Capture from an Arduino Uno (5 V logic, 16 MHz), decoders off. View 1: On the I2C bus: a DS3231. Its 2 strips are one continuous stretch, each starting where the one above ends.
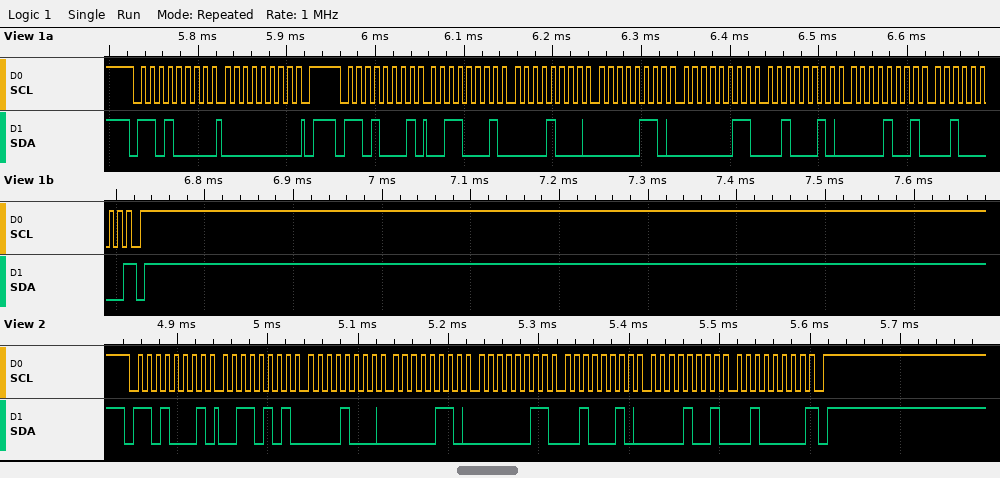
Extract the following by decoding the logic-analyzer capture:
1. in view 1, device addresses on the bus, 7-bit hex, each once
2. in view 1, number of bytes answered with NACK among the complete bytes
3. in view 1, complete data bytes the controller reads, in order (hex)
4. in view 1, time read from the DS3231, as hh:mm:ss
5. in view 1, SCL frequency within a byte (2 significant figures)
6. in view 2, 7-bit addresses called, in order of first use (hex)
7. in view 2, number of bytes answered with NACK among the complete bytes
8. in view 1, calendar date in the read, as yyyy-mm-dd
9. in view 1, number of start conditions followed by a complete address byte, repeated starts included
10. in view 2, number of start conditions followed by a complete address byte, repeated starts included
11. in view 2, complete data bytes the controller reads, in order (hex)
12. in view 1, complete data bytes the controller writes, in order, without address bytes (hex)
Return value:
0x68
1
31 08 06 03 22 09 20
06:08:31
100 kHz
0x68
1
2020-09-22
2
1
35 08 06 03 22 09 20
00
